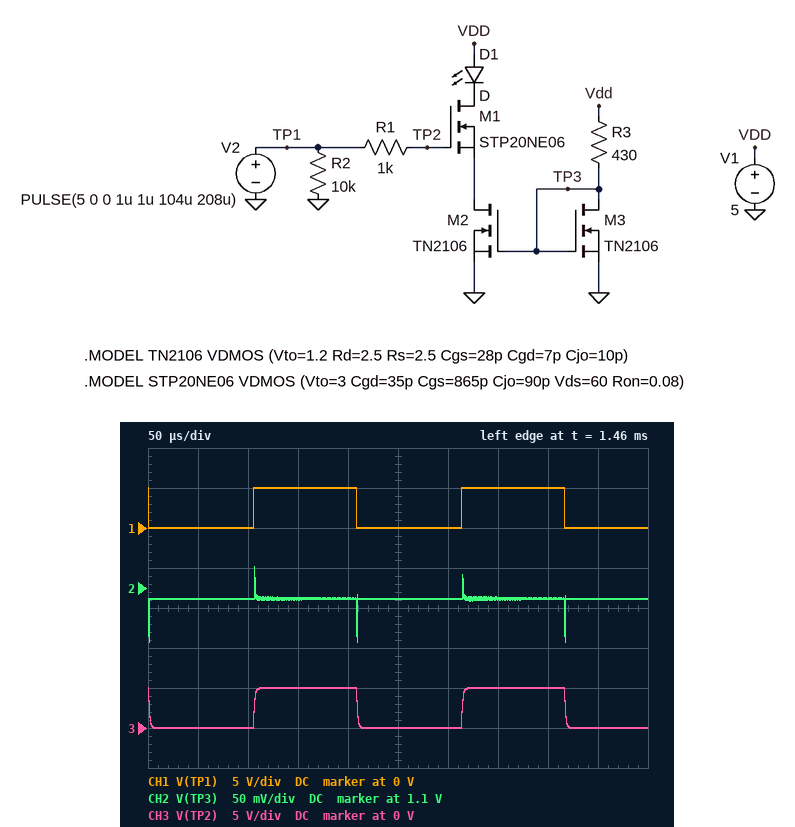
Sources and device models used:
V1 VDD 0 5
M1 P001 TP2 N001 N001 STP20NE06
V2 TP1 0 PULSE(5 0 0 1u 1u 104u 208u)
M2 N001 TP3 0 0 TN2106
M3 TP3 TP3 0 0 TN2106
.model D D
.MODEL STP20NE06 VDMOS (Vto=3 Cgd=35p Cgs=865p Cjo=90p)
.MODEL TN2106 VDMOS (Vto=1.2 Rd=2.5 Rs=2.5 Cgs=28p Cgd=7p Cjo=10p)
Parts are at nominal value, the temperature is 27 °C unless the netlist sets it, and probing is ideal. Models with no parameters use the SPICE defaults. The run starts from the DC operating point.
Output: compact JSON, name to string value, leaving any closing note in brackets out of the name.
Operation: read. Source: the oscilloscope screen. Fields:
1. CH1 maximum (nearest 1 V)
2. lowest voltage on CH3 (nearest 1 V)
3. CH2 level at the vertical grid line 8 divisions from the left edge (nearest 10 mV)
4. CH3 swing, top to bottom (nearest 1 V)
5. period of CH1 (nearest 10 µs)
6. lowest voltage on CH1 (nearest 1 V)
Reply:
{"CH1 maximum": "5 V", "lowest voltage on CH3": "0 V", "CH2 level at the vertical grid line 8 divisions from the left edge": "1.09 V", "CH3 swing, top to bottom": "5 V", "period of CH1": "210 µs", "lowest voltage on CH1": "0 V"}
